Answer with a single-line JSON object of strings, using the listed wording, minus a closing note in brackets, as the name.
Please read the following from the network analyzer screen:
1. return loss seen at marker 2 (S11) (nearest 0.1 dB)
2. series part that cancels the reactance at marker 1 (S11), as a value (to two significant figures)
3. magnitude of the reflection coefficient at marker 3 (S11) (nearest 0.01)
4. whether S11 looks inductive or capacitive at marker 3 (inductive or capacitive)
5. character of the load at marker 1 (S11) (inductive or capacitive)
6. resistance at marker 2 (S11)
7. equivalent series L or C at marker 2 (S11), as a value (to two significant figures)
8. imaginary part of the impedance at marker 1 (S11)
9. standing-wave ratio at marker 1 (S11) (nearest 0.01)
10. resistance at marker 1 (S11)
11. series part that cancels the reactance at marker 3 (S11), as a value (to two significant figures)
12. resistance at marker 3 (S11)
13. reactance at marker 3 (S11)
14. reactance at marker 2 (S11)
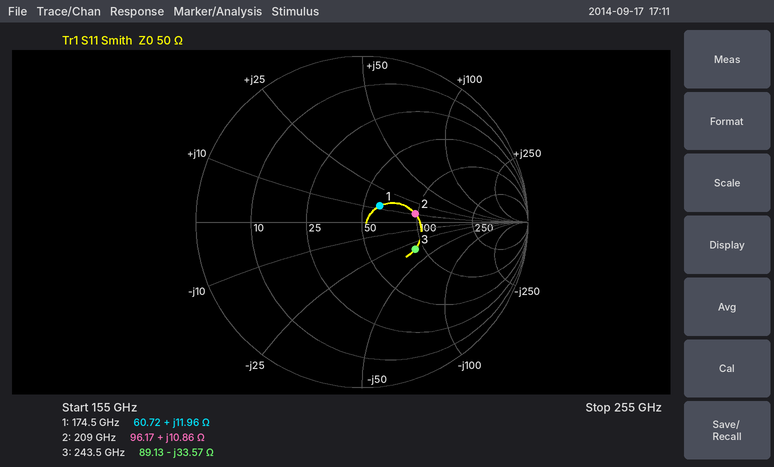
{"return loss seen at marker 2 (S11)": "9.8 dB", "series part that cancels the reactance at marker 1 (S11), as a value": "76 fF", "magnitude of the reflection coefficient at marker 3 (S11)": "0.36", "whether S11 looks inductive or capacitive at marker 3": "capacitive", "character of the load at marker 1 (S11)": "inductive", "resistance at marker 2": "96.17 Ω", "equivalent series L or C at marker 2 (S11), as a value": "8.3 pH", "imaginary part of the impedance at marker 1": "+11.96 Ω", "standing-wave ratio at marker 1 (S11)": "1.34", "resistance at marker 1": "60.72 Ω", "series part that cancels the reactance at marker 3 (S11), as a value": "22 pH", "resistance at marker 3": "89.13 Ω", "reactance at marker 3": "-33.57 Ω", "reactance at marker 2": "+10.86 Ω"}
